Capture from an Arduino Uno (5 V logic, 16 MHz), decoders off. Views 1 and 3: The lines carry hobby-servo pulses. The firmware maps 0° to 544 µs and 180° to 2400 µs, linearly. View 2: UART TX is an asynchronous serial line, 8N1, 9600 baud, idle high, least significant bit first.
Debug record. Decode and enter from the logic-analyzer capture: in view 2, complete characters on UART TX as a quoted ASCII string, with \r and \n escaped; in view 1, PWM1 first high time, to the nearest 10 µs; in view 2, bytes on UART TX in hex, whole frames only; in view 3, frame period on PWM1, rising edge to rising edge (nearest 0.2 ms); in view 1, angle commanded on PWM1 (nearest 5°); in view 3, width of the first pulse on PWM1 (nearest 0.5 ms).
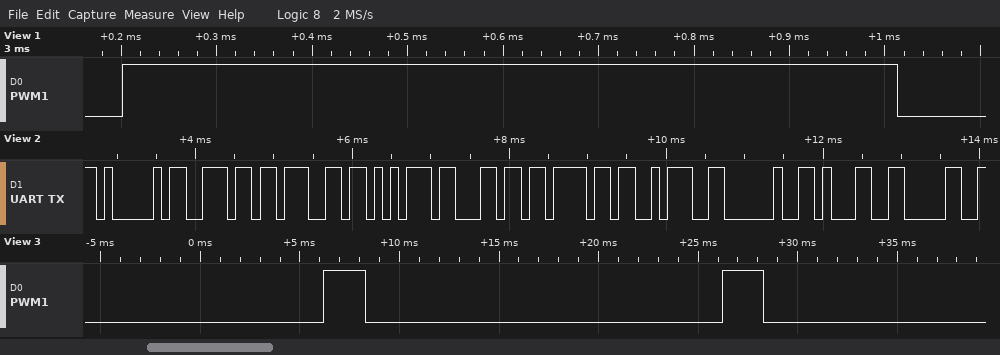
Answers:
"Angulo: 10"
810 µs
41 6E 67 75 6C 6F 3A 20 31 30
20.0 ms
25°
2.0 ms
